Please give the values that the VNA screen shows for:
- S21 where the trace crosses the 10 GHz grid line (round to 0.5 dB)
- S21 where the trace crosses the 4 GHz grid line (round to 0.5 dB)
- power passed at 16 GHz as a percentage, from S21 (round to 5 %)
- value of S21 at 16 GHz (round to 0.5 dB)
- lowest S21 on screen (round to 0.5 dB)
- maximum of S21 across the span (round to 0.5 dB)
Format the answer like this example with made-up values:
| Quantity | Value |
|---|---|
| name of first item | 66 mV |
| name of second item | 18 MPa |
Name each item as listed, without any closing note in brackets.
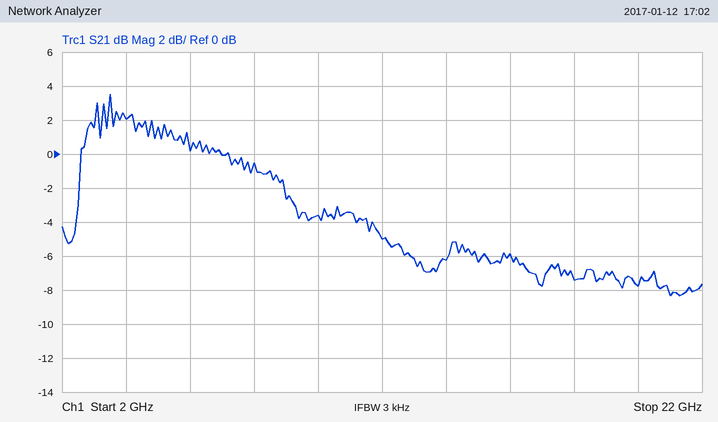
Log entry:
| Quantity | Value |
|---|---|
| S21 where the trace crosses the 10 GHz grid line | -3.5 dB |
| S21 where the trace crosses the 4 GHz grid line | 2.0 dB |
| power passed at 16 GHz as a percentage, from S21 | 25 % |
| value of S21 at 16 GHz | -6.0 dB |
| lowest S21 on screen | -8.5 dB |
| maximum of S21 across the span | 3.5 dB |
